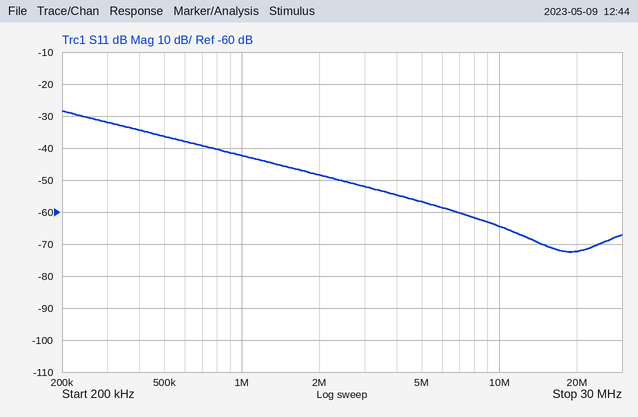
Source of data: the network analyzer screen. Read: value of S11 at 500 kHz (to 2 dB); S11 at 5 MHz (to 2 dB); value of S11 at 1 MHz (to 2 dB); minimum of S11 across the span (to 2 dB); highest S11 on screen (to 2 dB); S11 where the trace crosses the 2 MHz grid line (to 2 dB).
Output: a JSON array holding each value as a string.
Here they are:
["-36 dB", "-56 dB", "-42 dB", "-72 dB", "-28 dB", "-48 dB"]
